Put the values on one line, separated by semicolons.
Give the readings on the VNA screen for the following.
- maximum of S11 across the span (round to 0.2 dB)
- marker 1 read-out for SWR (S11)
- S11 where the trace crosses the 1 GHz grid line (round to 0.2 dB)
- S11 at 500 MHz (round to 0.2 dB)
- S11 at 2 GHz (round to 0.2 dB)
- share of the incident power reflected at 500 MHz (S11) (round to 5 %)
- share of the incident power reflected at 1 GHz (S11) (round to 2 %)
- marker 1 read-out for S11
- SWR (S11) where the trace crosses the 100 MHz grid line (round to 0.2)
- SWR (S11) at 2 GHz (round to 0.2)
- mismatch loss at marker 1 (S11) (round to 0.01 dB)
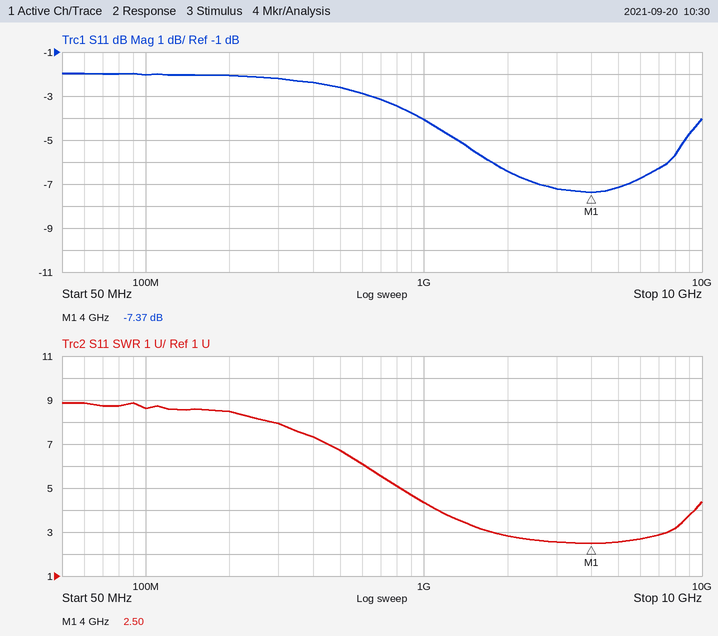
-2.0 dB; 2.50; -4.0 dB; -2.6 dB; -6.4 dB; 55 %; 40 %; -7.37 dB; 8.6; 2.8; 0.88 dB
